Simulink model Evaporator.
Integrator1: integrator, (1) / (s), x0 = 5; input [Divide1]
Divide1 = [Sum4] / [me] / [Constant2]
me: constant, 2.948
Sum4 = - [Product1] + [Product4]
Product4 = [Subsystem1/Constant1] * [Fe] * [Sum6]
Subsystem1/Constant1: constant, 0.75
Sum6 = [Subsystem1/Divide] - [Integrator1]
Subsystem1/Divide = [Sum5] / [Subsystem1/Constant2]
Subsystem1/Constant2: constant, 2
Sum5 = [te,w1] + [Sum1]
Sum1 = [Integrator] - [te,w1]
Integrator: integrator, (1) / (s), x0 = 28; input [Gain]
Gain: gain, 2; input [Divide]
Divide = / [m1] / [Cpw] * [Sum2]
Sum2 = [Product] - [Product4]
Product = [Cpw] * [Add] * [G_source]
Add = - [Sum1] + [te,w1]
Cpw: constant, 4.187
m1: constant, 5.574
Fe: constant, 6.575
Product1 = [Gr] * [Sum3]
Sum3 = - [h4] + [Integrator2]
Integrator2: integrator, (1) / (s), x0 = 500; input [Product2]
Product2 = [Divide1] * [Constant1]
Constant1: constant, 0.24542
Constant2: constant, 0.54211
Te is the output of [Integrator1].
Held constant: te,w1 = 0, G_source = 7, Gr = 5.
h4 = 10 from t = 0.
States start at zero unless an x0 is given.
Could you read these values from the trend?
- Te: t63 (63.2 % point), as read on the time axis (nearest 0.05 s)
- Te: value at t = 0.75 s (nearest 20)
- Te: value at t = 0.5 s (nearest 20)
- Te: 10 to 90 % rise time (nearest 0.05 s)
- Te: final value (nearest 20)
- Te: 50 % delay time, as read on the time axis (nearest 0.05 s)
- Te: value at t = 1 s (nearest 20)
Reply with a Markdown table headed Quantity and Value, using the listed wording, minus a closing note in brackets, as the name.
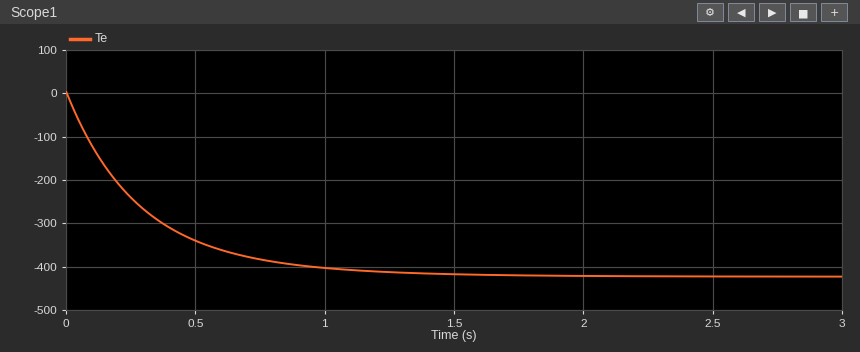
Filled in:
| Quantity | Value |
|---|---|
| Te: t63 (63.2 % point), as read on the time axis | 0.30 s |
| Te: value at t = 0.75 s | -380 |
| Te: value at t = 0.5 s | -340 |
| Te: 10 to 90 % rise time | 0.70 s |
| Te: final value | -420 |
| Te: 50 % delay time, as read on the time axis | 0.20 s |
| Te: value at t = 1 s | -400 |
